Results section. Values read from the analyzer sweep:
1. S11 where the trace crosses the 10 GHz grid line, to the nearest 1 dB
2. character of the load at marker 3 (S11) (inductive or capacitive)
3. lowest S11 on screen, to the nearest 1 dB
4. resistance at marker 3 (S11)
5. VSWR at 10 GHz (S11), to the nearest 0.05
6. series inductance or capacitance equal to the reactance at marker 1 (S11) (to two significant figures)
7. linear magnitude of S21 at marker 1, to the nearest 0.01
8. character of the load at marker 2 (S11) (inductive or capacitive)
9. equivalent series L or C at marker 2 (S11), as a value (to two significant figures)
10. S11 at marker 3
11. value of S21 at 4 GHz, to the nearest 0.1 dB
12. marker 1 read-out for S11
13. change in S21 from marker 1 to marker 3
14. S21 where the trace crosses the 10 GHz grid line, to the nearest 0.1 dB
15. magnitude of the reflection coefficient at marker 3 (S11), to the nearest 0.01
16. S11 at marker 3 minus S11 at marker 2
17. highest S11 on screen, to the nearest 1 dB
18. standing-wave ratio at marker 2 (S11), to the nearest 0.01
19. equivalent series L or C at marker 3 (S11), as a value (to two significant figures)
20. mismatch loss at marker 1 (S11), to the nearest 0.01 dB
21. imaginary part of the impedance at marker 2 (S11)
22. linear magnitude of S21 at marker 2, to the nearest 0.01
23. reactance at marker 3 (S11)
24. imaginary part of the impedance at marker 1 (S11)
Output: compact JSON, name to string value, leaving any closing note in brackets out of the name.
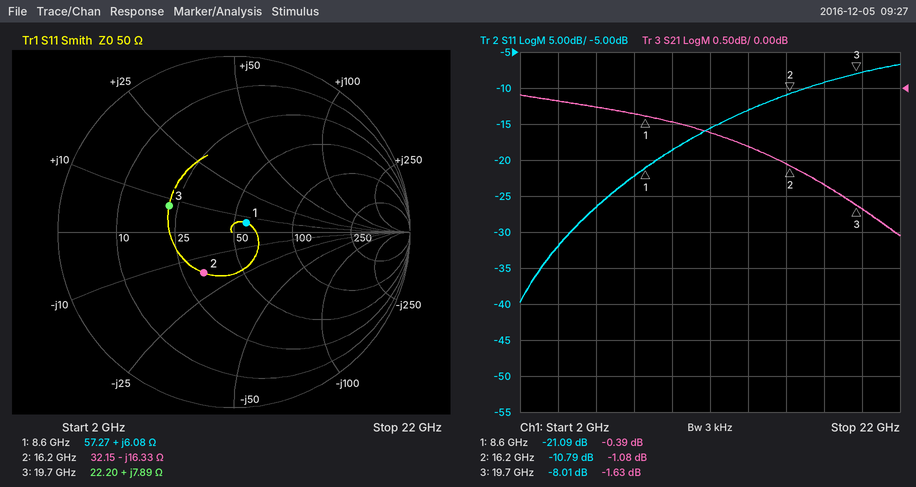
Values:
{"S11 where the trace crosses the 10 GHz grid line, to the nearest 1 dB": "-19 dB", "character of the load at marker 3 (S11)": "inductive", "lowest S11 on screen, to the nearest 1 dB": "-40 dB", "resistance at marker 3": "22.20 Ω", "VSWR at 10 GHz (S11), to the nearest 0.05": "1.25", "series inductance or capacitance equal to the reactance at marker 1 (S11)": "110 pH", "linear magnitude of S21 at marker 1, to the nearest 0.01": "0.96", "character of the load at marker 2 (S11)": "capacitive", "equivalent series L or C at marker 2 (S11), as a value": "600 fF", "S11 at marker 3": "-8.01 dB", "value of S21 at 4 GHz, to the nearest 0.1 dB": "-0.2 dB", "marker 1 read-out for S11": "-21.09 dB", "change in S21 from marker 1 to marker 3": "-1.24 dB", "S21 where the trace crosses the 10 GHz grid line, to the nearest 0.1 dB": "-0.5 dB", "magnitude of the reflection coefficient at marker 3 (S11), to the nearest 0.01": "0.40", "S11 at marker 3 minus S11 at marker 2": "2.78 dB", "highest S11 on screen, to the nearest 1 dB": "-7 dB", "standing-wave ratio at marker 2 (S11), to the nearest 0.01": "1.81", "equivalent series L or C at marker 3 (S11), as a value": "64 pH", "mismatch loss at marker 1 (S11), to the nearest 0.01 dB": "0.03 dB", "imaginary part of the impedance at marker 2": "-16.33 Ω", "linear magnitude of S21 at marker 2, to the nearest 0.01": "0.88", "reactance at marker 3": "+7.89 Ω", "imaginary part of the impedance at marker 1": "+6.08 Ω"}
